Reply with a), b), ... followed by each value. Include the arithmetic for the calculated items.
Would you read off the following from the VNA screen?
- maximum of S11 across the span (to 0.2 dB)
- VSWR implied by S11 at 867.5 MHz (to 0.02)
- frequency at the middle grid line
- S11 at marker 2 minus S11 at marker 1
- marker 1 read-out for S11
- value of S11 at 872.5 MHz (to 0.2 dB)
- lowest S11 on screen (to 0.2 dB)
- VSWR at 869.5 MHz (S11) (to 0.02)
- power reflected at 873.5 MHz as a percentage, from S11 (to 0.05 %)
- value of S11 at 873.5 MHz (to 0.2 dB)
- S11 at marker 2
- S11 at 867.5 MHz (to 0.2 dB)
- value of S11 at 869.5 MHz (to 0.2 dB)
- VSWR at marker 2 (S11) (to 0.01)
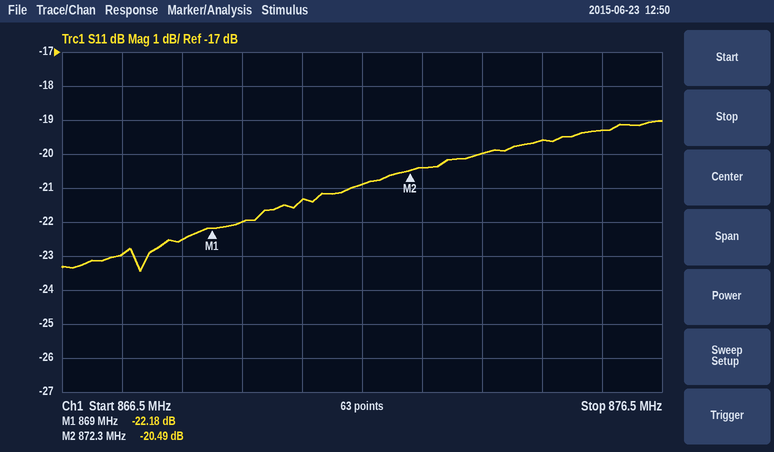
a) -19.0 dB
b) |Γ| = 10^(-23/20) = 0.0708; VSWR = (1 + 0.0708)/(1 − 0.0708) ≈ 1.15, so 1.16 to the nearest 0.02
c) 871.5 MHz
d) -20.49 − (-22.18) = 1.69 dB
e) -22.18 dB
f) -20.4 dB
g) -23.4 dB
h) |Γ| = 10^(-22/20) = 0.0794; VSWR = (1 + 0.0794)/(1 − 0.0794) ≈ 1.17, so 1.18 to the nearest 0.02
i) 10^(-20/10) ≈ 1.00 %
j) -20.0 dB
k) -20.49 dB
l) -23.0 dB
m) -22.0 dB
n) (1 + 0.0945)/(1 − 0.0945) ≈ 1.21
